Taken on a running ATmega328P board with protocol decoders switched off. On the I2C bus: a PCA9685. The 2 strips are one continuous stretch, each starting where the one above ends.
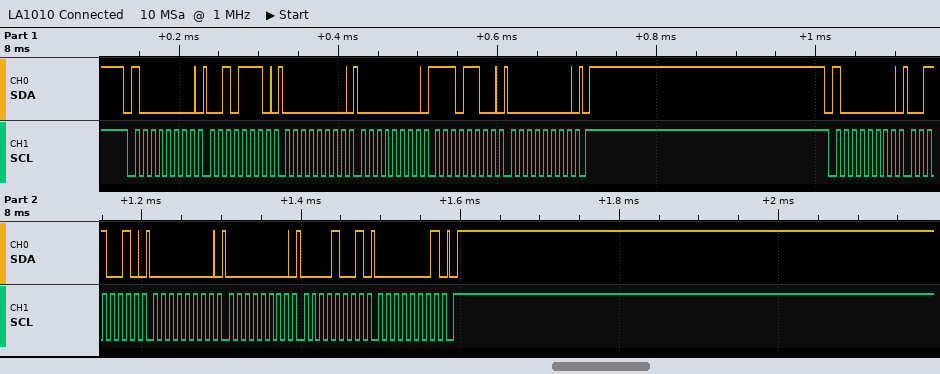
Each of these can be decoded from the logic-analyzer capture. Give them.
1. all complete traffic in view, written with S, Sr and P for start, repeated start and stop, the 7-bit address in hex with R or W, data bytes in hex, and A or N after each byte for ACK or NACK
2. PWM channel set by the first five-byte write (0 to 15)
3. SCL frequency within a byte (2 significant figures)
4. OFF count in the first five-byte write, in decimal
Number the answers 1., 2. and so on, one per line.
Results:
1. S 40W A 2E A 00 A 00 A EC A 00 A P S 40W A 32 A 00 A 00 A 09 A 01 A P
2. 10
3. 100 kHz
4. 236
